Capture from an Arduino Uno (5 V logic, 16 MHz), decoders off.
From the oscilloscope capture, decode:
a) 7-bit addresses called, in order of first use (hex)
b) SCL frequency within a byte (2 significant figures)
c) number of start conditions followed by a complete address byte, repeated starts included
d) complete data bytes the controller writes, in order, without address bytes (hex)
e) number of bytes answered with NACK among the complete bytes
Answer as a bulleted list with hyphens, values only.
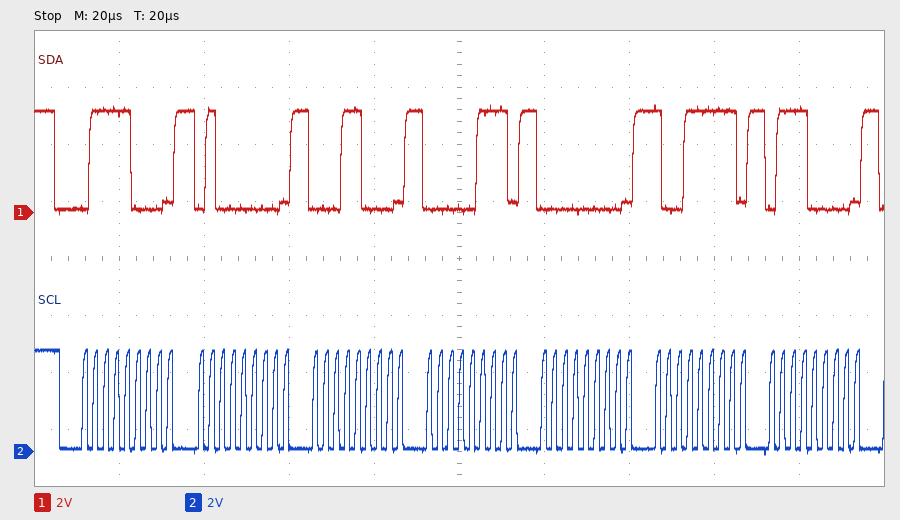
- 0x3C
- 400 kHz
- 1
- 40 18 07 00 9F 70
- 0
